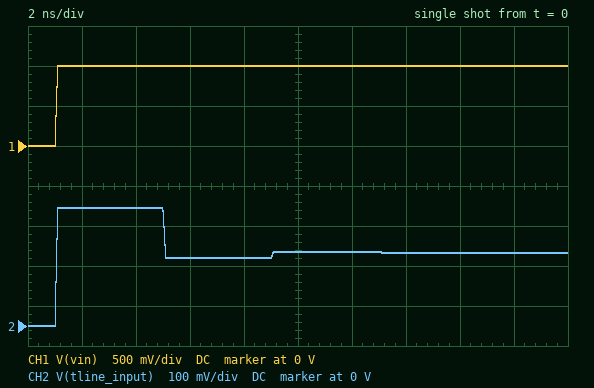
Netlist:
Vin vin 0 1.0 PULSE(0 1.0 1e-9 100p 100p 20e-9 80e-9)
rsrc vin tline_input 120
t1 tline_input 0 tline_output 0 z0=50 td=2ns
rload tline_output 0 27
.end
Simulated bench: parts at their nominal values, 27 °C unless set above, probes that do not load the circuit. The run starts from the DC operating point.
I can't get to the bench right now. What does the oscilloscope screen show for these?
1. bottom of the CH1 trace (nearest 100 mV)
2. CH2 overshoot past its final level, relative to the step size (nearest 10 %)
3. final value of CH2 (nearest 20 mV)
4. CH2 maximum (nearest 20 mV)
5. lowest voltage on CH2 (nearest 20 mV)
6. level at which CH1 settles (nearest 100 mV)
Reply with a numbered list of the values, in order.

1. 0 V
2. 60 %
3. 180 mV
4. 300 mV
5. 0 V
6. 1.0 V
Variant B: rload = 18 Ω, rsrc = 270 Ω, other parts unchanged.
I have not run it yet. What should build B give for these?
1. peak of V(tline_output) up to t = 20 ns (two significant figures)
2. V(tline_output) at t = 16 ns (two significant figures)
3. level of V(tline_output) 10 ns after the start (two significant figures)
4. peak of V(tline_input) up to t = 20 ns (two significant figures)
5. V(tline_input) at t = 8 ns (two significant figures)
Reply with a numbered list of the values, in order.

1. 83 mV
2. 62 mV
3. 56 mV
4. 160 mV
5. 32 mV
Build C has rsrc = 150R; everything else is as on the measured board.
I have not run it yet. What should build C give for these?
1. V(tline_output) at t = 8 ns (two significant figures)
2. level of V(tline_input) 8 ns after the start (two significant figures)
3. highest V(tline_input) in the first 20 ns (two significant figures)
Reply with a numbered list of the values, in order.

1. 150 mV
2. 140 mV
3. 250 mV
